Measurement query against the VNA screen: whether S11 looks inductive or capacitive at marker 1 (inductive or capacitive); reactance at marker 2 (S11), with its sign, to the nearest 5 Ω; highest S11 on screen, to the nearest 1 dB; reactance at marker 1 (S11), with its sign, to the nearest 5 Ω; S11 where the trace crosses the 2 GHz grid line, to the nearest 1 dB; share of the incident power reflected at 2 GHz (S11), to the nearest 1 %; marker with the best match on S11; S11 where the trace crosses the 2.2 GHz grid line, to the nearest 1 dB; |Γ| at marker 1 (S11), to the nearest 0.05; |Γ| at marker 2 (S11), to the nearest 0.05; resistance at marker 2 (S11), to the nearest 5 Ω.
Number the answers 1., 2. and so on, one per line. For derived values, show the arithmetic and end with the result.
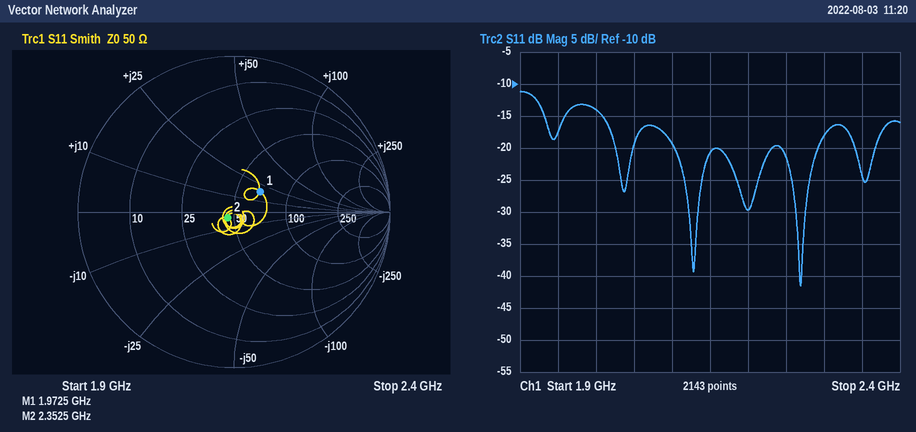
1. inductive
2. -5 Ω
3. -11 dB
4. +20 Ω
5. -14 dB
6. 10^(-14/10) ≈ 4 %
7. marker 2
8. -30 dB
9. 0.20
10. 0.05
11. 45 Ω
